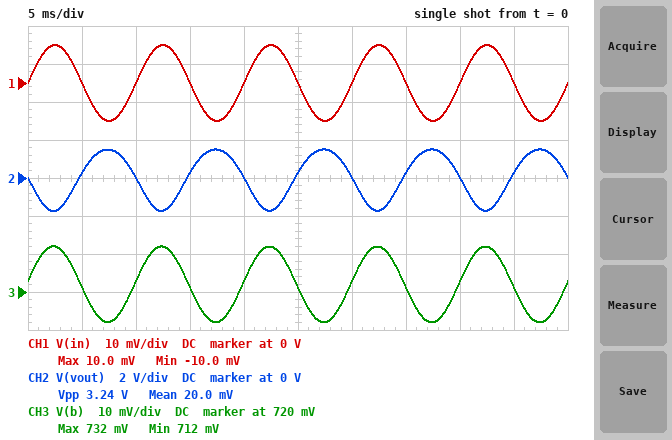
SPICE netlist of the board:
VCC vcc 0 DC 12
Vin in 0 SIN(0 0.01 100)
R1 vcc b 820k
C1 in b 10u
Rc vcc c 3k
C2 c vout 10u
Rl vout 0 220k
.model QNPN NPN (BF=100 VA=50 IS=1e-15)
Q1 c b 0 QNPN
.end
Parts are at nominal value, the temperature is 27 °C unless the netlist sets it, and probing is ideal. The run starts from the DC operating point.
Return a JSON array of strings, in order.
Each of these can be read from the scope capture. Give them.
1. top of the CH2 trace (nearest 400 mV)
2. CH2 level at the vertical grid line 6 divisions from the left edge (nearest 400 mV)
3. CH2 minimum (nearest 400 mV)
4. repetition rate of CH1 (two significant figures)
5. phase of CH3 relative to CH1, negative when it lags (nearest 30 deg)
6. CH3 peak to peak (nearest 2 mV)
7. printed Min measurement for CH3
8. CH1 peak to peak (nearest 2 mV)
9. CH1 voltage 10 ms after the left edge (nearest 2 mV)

["1.6 V", "0 V", "-1.6 V", "100 Hz", "0 deg", "20 mV", "712 mV", "20 mV", "0 V"]
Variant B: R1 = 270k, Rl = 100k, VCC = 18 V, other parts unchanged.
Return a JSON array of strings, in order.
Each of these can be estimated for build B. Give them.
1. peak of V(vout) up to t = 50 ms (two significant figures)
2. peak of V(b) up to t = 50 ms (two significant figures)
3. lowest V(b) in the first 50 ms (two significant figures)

["5.4 V", "760 mV", "750 mV"]
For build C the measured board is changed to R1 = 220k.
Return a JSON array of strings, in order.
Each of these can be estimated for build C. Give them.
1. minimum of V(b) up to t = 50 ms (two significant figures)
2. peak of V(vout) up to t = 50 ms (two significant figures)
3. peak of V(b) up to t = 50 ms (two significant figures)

["740 mV", "3.6 V", "750 mV"]
